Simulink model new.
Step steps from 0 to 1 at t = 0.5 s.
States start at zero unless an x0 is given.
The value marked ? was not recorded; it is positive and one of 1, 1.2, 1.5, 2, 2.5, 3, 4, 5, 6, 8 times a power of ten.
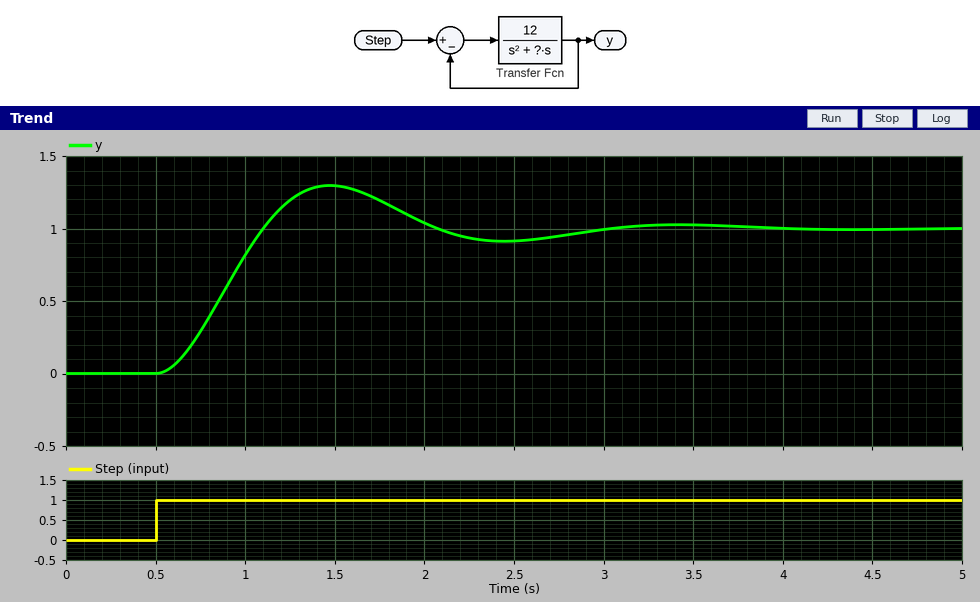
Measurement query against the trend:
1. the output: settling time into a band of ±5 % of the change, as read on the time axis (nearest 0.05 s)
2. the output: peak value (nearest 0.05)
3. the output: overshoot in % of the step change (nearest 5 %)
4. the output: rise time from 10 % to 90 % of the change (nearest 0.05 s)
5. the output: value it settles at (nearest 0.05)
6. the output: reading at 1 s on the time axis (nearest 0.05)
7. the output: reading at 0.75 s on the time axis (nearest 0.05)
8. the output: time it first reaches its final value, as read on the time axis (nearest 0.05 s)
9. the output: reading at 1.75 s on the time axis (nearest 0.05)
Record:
2.75 s
1.30
30 %
0.40 s
1.00
0.80
0.30
1.10 s
1.20
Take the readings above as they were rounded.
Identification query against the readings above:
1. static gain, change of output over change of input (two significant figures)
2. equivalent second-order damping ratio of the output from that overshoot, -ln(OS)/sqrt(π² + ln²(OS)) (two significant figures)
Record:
1.0
0.36
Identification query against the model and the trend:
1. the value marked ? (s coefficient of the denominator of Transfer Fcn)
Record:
2.5
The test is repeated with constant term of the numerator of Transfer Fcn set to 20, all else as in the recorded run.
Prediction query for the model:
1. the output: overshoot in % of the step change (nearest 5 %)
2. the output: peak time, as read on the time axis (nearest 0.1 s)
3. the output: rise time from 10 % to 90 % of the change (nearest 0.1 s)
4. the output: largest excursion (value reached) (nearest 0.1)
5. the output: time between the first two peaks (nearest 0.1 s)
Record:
40 %
1.2 s
0.3 s
1.4
1.5 s
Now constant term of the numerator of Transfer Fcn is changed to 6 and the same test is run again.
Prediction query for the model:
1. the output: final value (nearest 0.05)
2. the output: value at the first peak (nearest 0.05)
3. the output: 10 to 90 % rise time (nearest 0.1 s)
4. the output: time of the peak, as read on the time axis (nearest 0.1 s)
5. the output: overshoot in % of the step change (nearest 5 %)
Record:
1.00
1.15
0.7 s
2.0 s
15 %
